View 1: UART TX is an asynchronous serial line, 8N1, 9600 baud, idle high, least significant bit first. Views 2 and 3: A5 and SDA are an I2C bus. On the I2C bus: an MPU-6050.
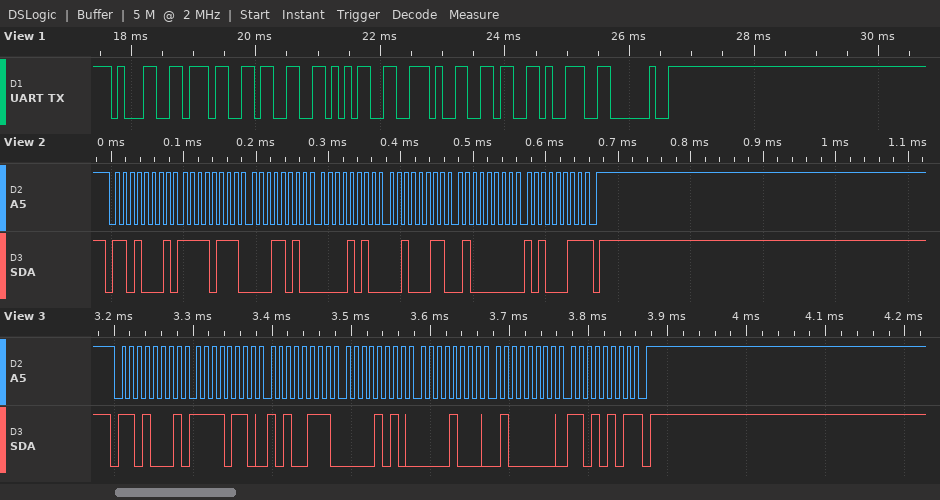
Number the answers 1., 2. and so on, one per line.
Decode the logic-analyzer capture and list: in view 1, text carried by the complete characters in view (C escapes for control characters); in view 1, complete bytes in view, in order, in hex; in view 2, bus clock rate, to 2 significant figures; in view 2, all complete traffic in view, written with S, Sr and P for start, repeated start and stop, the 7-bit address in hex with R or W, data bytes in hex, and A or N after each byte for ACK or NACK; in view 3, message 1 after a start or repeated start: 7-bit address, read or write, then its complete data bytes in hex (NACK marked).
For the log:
1. "1735.69 "
2. 31 37 33 35 2E 36 39 20
3. 100 kHz
4. S 68R A F7 A 1A A 0A A 23 A 40 A A3 N P
5. 0x68 read: F6 A7 0A 08 40 D5 NACK
